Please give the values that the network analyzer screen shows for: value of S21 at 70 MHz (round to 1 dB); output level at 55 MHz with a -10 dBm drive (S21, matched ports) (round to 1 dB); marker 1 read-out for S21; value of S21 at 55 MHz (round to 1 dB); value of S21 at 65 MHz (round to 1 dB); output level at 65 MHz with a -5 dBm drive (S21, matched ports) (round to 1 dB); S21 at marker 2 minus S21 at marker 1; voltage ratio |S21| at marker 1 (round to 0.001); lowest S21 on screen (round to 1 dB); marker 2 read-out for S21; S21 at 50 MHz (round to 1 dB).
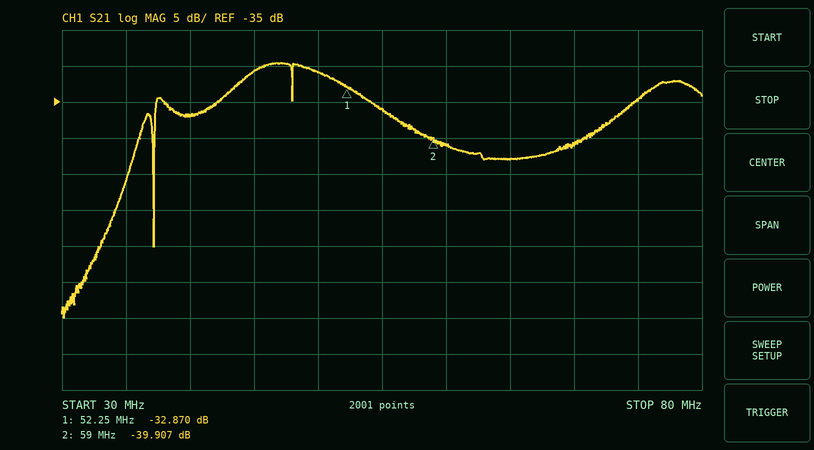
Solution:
-41 dB
-46 dBm
-32.870 dB
-36 dB
-43 dB
-48 dBm
-7.037 dB
0.023
-65 dB
-39.907 dB
-31 dB
